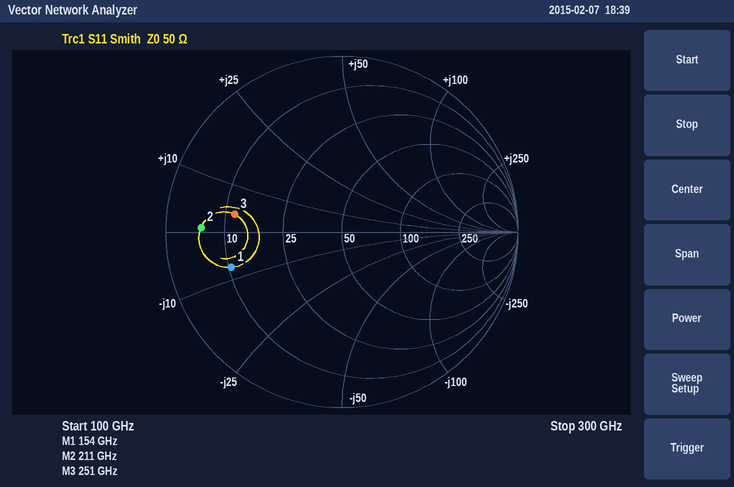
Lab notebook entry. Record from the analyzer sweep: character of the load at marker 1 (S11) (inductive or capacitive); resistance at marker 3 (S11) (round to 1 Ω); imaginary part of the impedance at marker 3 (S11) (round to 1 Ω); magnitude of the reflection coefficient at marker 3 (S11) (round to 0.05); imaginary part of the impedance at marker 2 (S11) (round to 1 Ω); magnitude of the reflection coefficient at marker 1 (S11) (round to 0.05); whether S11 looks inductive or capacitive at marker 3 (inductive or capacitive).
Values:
capacitive
12 Ω
+4 Ω
0.60
+1 Ω
0.65
inductive
